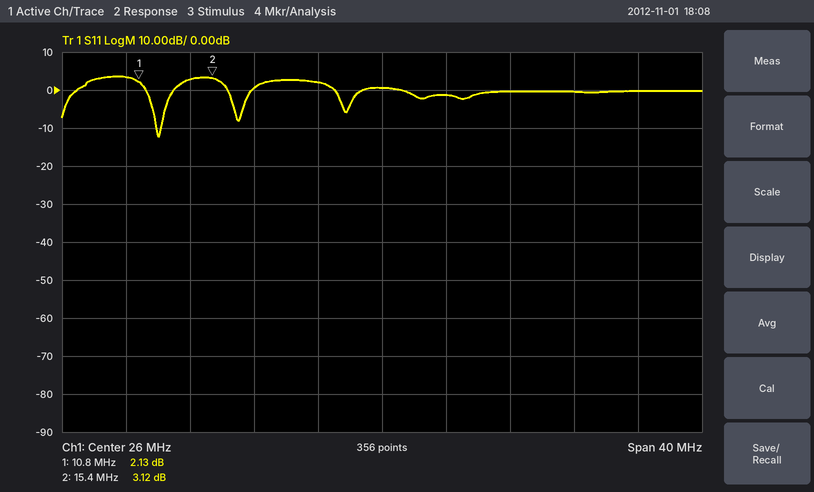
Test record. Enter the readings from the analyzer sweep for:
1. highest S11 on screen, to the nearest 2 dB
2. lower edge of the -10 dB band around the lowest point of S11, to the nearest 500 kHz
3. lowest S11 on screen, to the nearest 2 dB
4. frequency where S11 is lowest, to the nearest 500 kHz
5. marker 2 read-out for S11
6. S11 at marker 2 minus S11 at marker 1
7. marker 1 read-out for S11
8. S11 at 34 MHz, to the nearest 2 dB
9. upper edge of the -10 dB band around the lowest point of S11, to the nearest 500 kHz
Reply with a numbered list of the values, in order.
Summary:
1. 4 dB
2. 12.0 MHz
3. -12 dB
4. 12.0 MHz
5. 3.12 dB
6. 0.99 dB
7. 2.13 dB
8. 0 dB
9. 12.0 MHz
